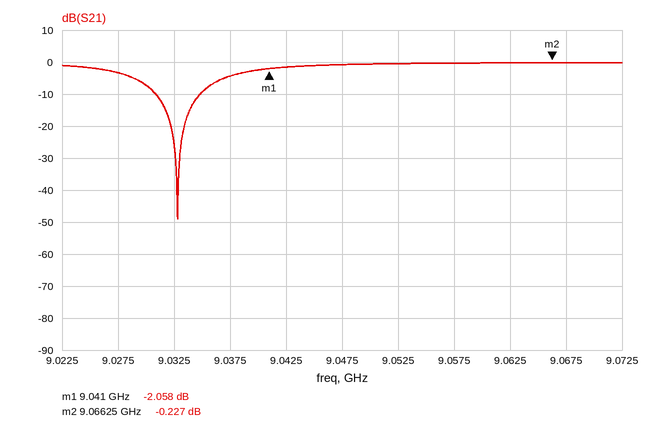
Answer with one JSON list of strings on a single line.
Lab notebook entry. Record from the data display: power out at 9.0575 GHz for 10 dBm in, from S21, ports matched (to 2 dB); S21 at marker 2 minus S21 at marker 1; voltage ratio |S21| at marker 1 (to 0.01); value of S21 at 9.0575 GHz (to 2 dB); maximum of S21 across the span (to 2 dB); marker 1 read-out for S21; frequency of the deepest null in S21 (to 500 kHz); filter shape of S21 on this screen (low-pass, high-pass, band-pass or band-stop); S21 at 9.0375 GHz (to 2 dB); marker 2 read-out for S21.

["10 dBm", "1.831 dB", "0.79", "0 dB", "0 dB", "-2.058 dB", "9.0330 GHz", "band-stop", "-4 dB", "-0.227 dB"]
